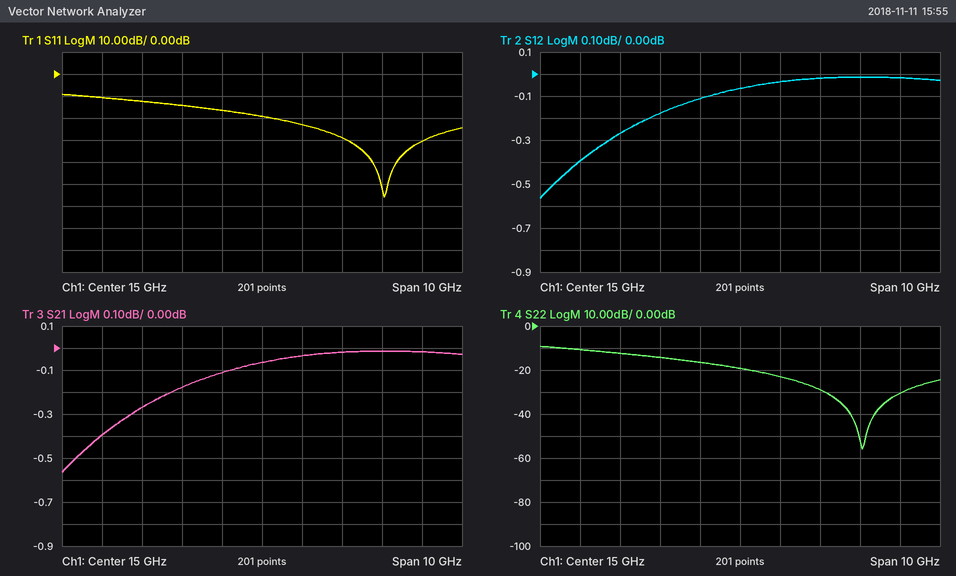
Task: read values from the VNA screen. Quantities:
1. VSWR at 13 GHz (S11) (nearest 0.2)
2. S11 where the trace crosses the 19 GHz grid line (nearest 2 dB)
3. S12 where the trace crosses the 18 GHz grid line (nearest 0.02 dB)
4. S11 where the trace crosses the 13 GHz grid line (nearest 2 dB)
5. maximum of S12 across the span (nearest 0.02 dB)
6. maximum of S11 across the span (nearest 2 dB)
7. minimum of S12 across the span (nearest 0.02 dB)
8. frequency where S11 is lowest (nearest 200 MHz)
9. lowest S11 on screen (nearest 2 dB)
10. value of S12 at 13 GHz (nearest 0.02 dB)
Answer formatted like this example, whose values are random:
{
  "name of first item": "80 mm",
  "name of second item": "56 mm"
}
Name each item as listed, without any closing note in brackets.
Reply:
{
  "VSWR at 13 GHz (S11)": "1.4",
  "S11 where the trace crosses the 19 GHz grid line": "-30 dB",
  "S12 where the trace crosses the 18 GHz grid line": "-0.02 dB",
  "S11 where the trace crosses the 13 GHz grid line": "-14 dB",
  "maximum of S12 across the span": "-0.02 dB",
  "maximum of S11 across the span": "-10 dB",
  "minimum of S12 across the span": "-0.56 dB",
  "frequency where S11 is lowest": "18.0 GHz",
  "lowest S11 on screen": "-56 dB",
  "value of S12 at 13 GHz": "-0.18 dB"
}
